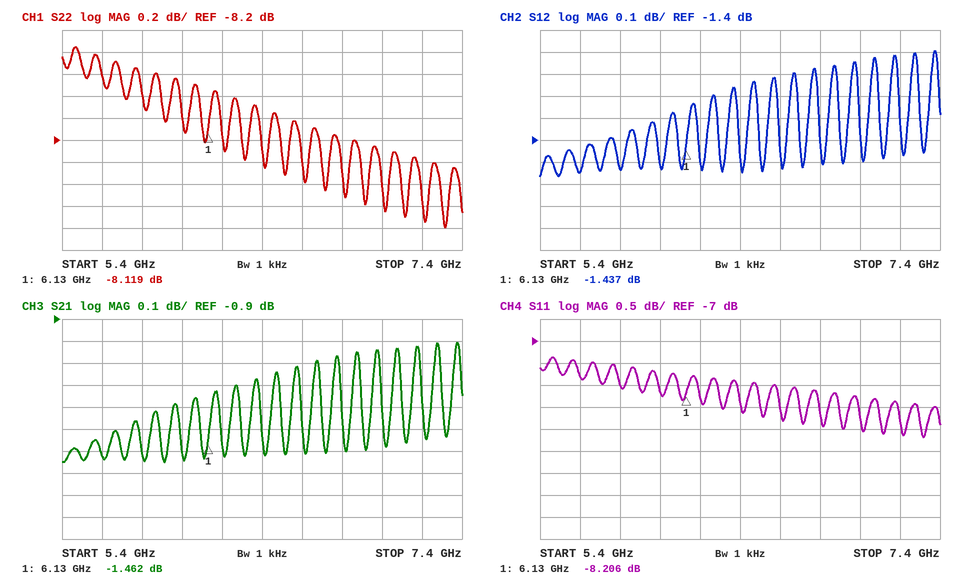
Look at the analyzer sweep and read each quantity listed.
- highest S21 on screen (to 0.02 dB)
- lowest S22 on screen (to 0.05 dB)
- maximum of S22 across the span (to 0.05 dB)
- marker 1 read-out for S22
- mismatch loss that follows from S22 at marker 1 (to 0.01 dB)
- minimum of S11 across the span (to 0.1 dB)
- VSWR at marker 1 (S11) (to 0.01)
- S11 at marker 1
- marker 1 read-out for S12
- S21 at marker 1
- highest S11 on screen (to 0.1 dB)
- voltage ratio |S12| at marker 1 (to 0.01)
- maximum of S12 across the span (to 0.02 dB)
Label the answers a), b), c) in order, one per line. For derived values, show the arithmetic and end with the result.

a) -1.00 dB
b) -9.00 dB
c) -7.35 dB
d) -8.119 dB
e) −10 log10(1 − 10^(-8.119/10)) ≈ 0.73 dB
f) -9.2 dB
g) (1 + 0.3888)/(1 − 0.3888) ≈ 2.27
h) -8.206 dB
i) -1.437 dB
j) -1.462 dB
k) -7.4 dB
l) 10^(-1.437/20) ≈ 0.85
m) -1.00 dB
